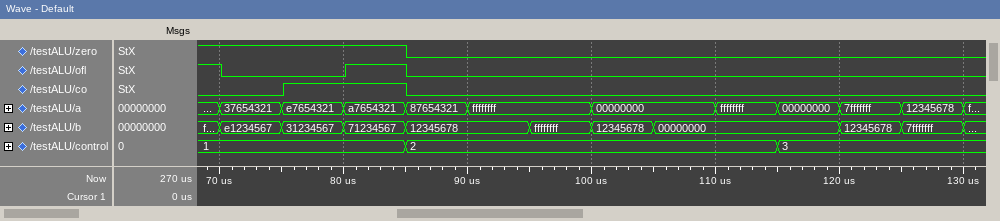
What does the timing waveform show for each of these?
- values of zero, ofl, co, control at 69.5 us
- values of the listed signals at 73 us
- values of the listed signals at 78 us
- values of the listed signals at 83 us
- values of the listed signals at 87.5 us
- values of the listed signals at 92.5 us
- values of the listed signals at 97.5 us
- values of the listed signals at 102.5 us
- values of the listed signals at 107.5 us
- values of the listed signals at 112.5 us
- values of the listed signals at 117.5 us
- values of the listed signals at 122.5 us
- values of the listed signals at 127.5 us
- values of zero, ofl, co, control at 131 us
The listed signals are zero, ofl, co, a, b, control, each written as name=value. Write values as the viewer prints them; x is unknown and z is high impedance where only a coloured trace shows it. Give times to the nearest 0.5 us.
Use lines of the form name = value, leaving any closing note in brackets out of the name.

values of zero, ofl, co, control at 69.5 us = zero=1, ofl=1, co=0, control=1
values of the listed signals at 73 us = zero=1, ofl=0, co=0, a=37654321, b=e1234567, control=1
values of the listed signals at 78 us = zero=1, ofl=0, co=1, a=e7654321, b=31234567, control=1
values of the listed signals at 83 us = zero=1, ofl=1, co=1, a=a7654321, b=71234567, control=1
values of the listed signals at 87.5 us = zero=0, ofl=0, co=0, a=87654321, b=12345678, control=2
values of the listed signals at 92.5 us = zero=0, ofl=0, co=0, a=ffffffff, b=12345678, control=2
values of the listed signals at 97.5 us = zero=0, ofl=0, co=0, a=ffffffff, b=ffffffff, control=2
values of the listed signals at 102.5 us = zero=0, ofl=0, co=0, a=00000000, b=12345678, control=2
values of the listed signals at 107.5 us = zero=0, ofl=0, co=0, a=00000000, b=00000000, control=2
values of the listed signals at 112.5 us = zero=0, ofl=0, co=0, a=ffffffff, b=00000000, control=2
values of the listed signals at 117.5 us = zero=0, ofl=0, co=0, a=00000000, b=00000000, control=3
values of the listed signals at 122.5 us = zero=0, ofl=0, co=0, a=7fffffff, b=12345678, control=3
values of the listed signals at 127.5 us = zero=0, ofl=0, co=0, a=12345678, b=7fffffff, control=3
values of zero, ofl, co, control at 131 us = zero=0, ofl=0, co=0, control=3
